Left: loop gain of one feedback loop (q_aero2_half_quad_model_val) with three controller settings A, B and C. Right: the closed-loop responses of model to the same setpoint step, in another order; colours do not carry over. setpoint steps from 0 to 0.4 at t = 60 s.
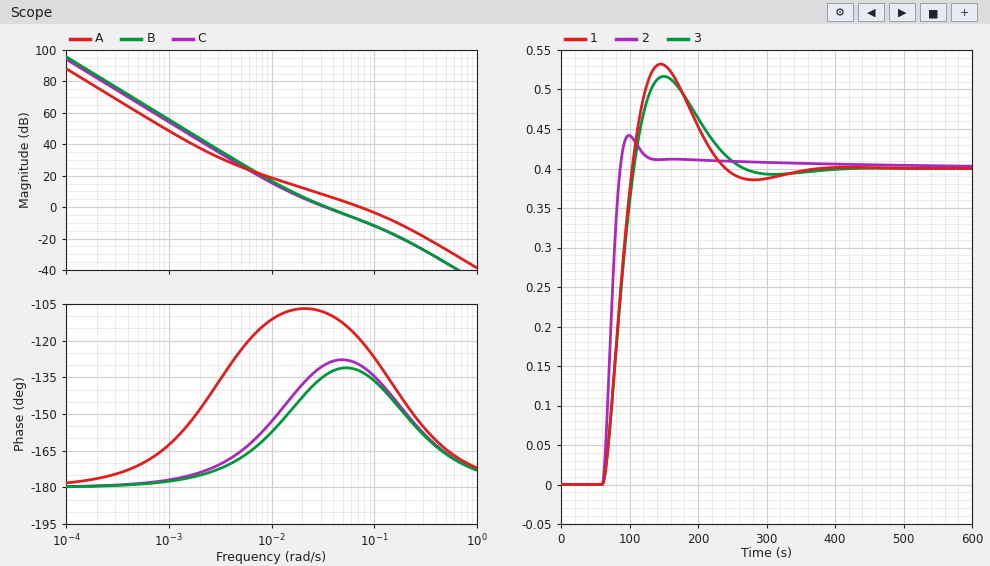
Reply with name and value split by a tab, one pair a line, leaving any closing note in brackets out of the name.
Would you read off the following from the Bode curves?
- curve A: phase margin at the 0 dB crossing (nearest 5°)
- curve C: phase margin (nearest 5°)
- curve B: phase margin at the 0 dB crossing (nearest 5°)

curve A: phase margin at the 0 dB crossing	60°
curve C: phase margin	50°
curve B: phase margin at the 0 dB crossing	45°
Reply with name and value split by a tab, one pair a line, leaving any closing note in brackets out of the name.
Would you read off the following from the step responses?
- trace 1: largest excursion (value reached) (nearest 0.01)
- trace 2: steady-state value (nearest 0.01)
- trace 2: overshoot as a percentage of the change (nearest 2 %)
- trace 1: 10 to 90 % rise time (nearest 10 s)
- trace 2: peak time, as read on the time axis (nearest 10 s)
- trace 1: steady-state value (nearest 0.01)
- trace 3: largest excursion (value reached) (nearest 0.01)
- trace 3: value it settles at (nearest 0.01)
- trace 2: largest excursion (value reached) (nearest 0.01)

trace 1: largest excursion (value reached)	0.53
trace 2: steady-state value	0.40
trace 2: overshoot as a percentage of the change	10 %
trace 1: 10 to 90 % rise time	30 s
trace 2: peak time, as read on the time axis	100 s
trace 1: steady-state value	0.40
trace 3: largest excursion (value reached)	0.52
trace 3: value it settles at	0.40
trace 2: largest excursion (value reached)	0.44
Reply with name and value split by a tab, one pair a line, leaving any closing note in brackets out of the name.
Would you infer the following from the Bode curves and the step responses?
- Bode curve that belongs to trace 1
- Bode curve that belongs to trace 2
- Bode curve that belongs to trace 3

Bode curve that belongs to trace 1	B
Bode curve that belongs to trace 2	A
Bode curve that belongs to trace 3	C
